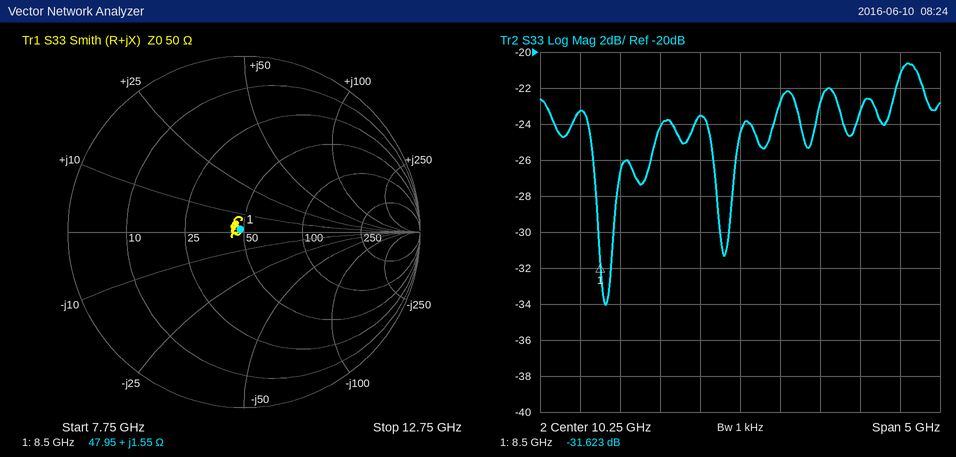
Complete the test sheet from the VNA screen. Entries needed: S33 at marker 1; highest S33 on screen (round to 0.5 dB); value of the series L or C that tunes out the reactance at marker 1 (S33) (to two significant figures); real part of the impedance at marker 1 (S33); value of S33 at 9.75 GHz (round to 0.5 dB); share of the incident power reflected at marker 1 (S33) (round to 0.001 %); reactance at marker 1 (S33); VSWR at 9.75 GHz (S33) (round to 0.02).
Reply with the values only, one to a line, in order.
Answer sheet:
-31.623 dB
-20.5 dB
12 pF
47.95 Ω
-23.5 dB
0.069 %
+1.55 Ω
1.14
